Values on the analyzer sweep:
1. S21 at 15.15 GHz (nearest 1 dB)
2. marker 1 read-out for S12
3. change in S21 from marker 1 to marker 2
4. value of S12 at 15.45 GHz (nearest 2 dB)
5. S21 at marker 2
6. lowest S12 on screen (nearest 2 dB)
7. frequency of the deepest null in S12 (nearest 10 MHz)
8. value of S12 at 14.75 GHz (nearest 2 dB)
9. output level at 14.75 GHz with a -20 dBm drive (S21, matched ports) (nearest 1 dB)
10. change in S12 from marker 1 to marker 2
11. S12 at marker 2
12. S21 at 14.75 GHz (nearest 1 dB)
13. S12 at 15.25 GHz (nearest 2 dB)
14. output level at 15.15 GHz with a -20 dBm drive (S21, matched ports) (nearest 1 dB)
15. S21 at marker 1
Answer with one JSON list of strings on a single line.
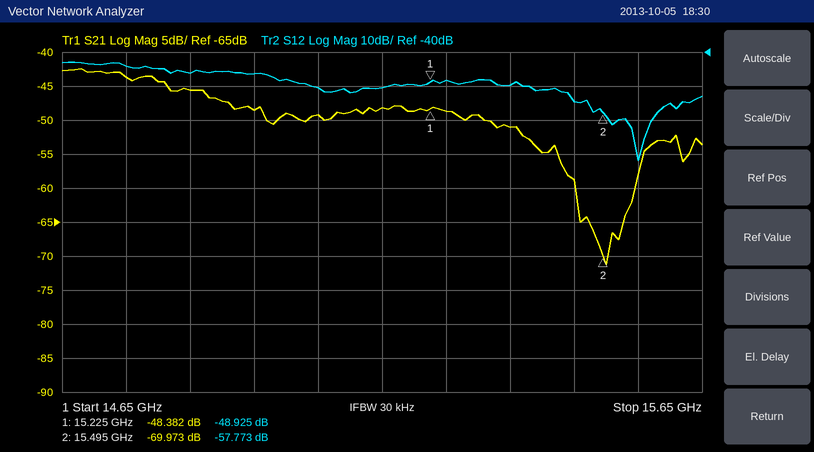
["-48 dB", "-48.925 dB", "-21.591 dB", "-54 dB", "-69.973 dB", "-72 dB", "15.55 GHz", "-44 dB", "-64 dBm", "-8.848 dB", "-57.773 dB", "-44 dB", "-48 dB", "-68 dBm", "-48.382 dB"]
